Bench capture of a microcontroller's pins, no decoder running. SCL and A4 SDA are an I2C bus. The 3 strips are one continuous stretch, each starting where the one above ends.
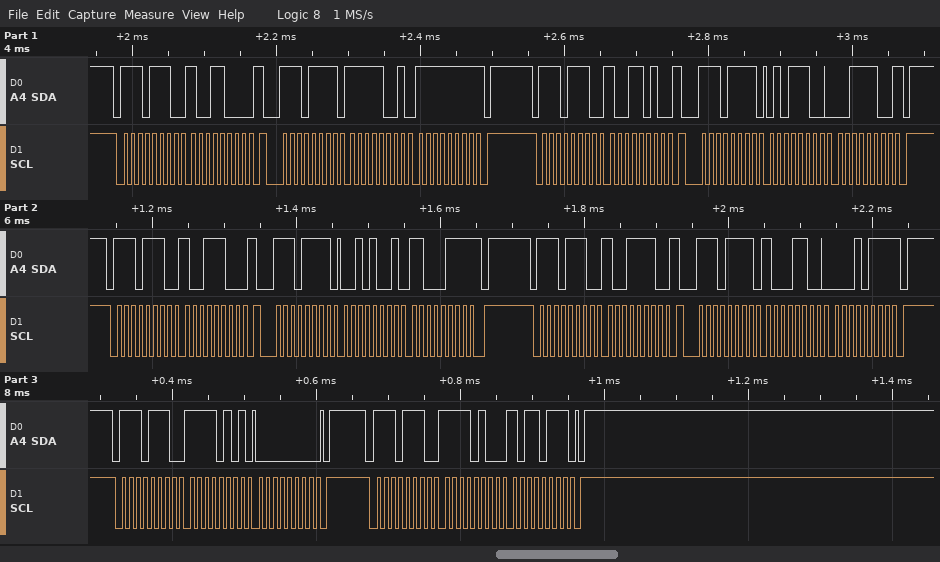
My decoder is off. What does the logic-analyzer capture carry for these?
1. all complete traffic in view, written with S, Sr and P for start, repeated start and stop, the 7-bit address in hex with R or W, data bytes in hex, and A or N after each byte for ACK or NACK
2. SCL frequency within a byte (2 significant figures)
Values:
S 77W A 98 A Sr 77R A F9 A FF N P S 77W A 9A A Sr 77R A 5C A 3C N P S 77W A 9C A Sr 77R A 29 A C7 N P S 77W A 9E A Sr 77R A 8C A 17 N P S 77W A F5 A 00 A P S 77W A F4 A B7 A P
100 kHz
